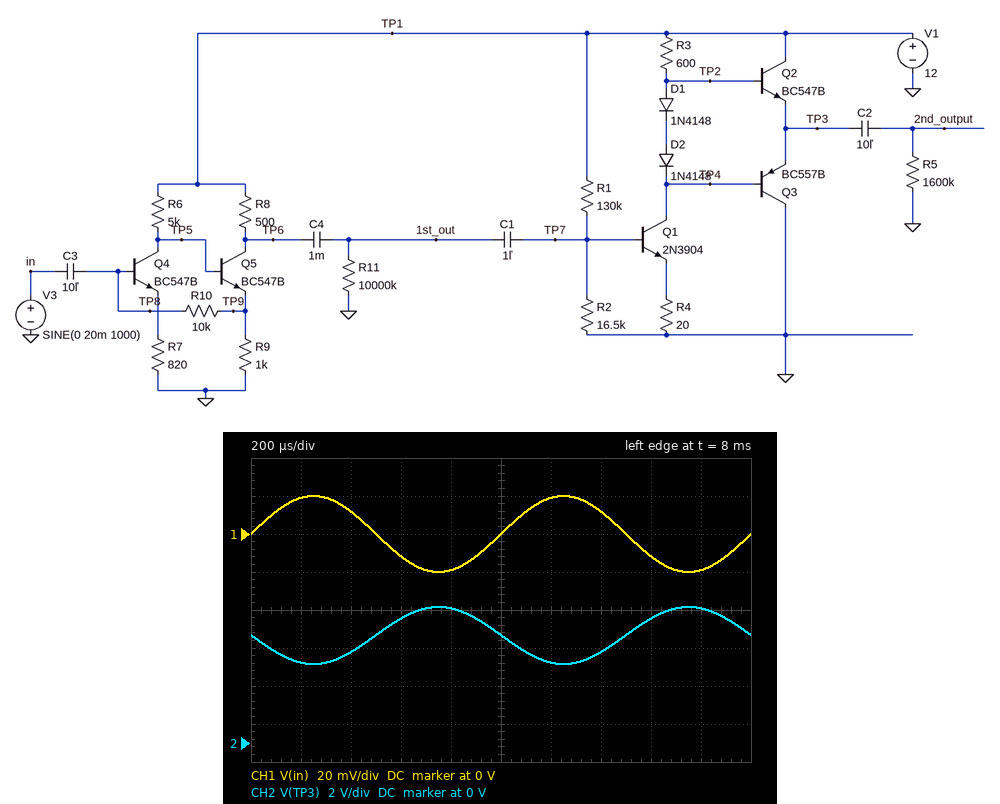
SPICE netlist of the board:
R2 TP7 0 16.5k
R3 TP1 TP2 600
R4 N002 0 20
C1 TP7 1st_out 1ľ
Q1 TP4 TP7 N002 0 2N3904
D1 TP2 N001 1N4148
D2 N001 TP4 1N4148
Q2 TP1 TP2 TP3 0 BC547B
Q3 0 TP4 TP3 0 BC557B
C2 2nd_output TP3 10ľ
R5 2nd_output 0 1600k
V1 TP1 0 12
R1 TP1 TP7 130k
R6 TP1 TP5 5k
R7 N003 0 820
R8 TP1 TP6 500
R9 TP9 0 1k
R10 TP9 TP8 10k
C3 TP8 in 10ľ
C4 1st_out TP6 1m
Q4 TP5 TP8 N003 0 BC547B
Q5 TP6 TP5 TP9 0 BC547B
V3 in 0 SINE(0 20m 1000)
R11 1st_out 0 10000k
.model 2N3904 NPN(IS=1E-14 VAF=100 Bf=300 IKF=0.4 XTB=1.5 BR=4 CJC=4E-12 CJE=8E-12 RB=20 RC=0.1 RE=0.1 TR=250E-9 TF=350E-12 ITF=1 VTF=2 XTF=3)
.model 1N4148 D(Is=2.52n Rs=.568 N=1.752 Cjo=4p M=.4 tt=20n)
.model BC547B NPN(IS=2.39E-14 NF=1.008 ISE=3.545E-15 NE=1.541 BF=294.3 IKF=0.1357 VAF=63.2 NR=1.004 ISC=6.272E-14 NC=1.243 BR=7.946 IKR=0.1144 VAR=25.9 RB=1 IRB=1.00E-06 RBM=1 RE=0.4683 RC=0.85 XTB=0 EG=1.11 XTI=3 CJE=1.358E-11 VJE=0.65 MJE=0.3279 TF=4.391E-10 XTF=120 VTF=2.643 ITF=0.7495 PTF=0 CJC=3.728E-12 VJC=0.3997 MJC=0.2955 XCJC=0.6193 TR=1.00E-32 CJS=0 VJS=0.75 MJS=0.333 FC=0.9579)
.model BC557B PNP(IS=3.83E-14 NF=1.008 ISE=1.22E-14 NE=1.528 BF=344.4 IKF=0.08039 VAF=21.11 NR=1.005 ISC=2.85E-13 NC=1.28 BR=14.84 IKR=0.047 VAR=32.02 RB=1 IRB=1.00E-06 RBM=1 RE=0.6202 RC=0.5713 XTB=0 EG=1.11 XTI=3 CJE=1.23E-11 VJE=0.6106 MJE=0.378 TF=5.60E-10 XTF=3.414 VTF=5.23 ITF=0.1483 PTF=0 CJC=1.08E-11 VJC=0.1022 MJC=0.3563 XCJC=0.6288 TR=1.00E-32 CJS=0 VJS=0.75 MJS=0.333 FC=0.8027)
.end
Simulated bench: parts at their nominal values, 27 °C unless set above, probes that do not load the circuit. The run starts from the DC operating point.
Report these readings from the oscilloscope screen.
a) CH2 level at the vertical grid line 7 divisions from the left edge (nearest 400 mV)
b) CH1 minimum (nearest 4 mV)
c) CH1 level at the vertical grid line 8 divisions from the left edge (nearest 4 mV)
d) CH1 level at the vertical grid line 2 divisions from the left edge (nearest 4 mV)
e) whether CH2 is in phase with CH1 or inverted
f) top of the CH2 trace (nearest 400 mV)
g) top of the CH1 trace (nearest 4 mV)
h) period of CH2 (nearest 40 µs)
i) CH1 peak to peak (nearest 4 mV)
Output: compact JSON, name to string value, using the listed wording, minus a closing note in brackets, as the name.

{"CH2 level at the vertical grid line 7 divisions from the left edge": "4.8 V", "CH1 minimum": "-20 mV", "CH1 level at the vertical grid line 8 divisions from the left edge": "-12 mV", "CH1 level at the vertical grid line 2 divisions from the left edge": "12 mV", "whether CH2 is in phase with CH1 or inverted": "inverted", "top of the CH2 trace": "7.2 V", "top of the CH1 trace": "20 mV", "period of CH2": "1.00 ms", "CH1 peak to peak": "40 mV"}
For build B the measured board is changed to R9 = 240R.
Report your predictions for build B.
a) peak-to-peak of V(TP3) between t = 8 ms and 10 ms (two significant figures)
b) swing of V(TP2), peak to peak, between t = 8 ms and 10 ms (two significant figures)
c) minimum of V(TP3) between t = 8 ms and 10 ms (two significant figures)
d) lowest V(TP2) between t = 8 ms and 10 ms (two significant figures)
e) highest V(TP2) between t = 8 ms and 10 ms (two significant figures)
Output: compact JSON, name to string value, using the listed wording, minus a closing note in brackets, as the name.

{"peak-to-peak of V(TP3) between t = 8 ms and 10 ms": "9.3 V", "swing of V(TP2), peak to peak, between t = 8 ms and 10 ms": "9.2 V", "minimum of V(TP3) between t = 8 ms and 10 ms": "1.2 V", "lowest V(TP2) between t = 8 ms and 10 ms": "1.9 V", "highest V(TP2) between t = 8 ms and 10 ms": "11 V"}
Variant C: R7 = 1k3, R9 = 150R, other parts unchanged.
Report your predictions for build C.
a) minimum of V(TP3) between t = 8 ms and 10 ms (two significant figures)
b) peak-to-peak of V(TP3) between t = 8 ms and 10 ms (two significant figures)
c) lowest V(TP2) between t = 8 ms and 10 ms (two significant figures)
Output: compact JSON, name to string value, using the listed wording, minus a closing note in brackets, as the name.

{"minimum of V(TP3) between t = 8 ms and 10 ms": "5.6 V", "peak-to-peak of V(TP3) between t = 8 ms and 10 ms": "180 mV", "lowest V(TP2) between t = 8 ms and 10 ms": "6.3 V"}
